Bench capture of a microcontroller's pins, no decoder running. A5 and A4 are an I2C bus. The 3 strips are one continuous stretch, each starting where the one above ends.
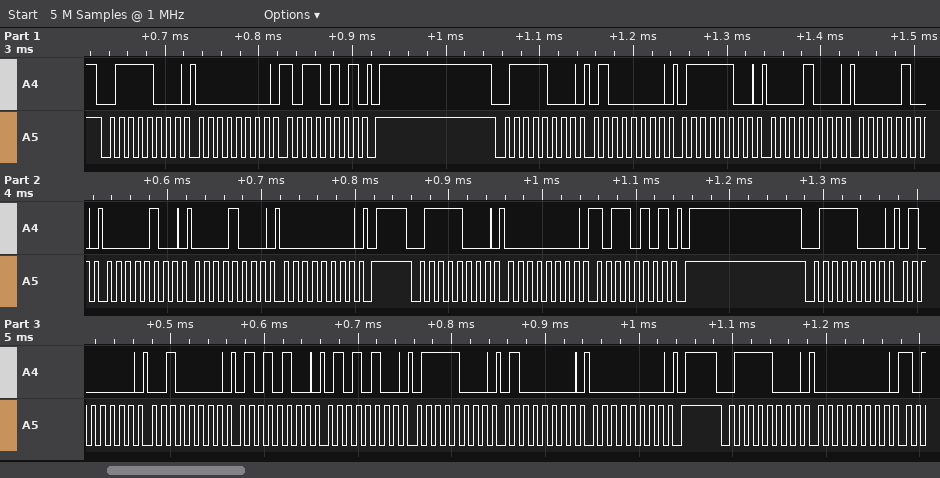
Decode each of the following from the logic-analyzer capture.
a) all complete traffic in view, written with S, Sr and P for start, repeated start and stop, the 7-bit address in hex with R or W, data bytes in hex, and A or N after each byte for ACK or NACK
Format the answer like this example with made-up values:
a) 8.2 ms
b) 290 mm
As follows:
a) S 3CW A 00 A B5 A P S 3CW A 40 A 7C A 08 A 04 A 04 A 08 A 00 A P S 3CW A 00 A B5 A P S 3CW A 40 A 20 A 54 A 54 A 78 A 40 A 00 A P S 3CW A 00 A
